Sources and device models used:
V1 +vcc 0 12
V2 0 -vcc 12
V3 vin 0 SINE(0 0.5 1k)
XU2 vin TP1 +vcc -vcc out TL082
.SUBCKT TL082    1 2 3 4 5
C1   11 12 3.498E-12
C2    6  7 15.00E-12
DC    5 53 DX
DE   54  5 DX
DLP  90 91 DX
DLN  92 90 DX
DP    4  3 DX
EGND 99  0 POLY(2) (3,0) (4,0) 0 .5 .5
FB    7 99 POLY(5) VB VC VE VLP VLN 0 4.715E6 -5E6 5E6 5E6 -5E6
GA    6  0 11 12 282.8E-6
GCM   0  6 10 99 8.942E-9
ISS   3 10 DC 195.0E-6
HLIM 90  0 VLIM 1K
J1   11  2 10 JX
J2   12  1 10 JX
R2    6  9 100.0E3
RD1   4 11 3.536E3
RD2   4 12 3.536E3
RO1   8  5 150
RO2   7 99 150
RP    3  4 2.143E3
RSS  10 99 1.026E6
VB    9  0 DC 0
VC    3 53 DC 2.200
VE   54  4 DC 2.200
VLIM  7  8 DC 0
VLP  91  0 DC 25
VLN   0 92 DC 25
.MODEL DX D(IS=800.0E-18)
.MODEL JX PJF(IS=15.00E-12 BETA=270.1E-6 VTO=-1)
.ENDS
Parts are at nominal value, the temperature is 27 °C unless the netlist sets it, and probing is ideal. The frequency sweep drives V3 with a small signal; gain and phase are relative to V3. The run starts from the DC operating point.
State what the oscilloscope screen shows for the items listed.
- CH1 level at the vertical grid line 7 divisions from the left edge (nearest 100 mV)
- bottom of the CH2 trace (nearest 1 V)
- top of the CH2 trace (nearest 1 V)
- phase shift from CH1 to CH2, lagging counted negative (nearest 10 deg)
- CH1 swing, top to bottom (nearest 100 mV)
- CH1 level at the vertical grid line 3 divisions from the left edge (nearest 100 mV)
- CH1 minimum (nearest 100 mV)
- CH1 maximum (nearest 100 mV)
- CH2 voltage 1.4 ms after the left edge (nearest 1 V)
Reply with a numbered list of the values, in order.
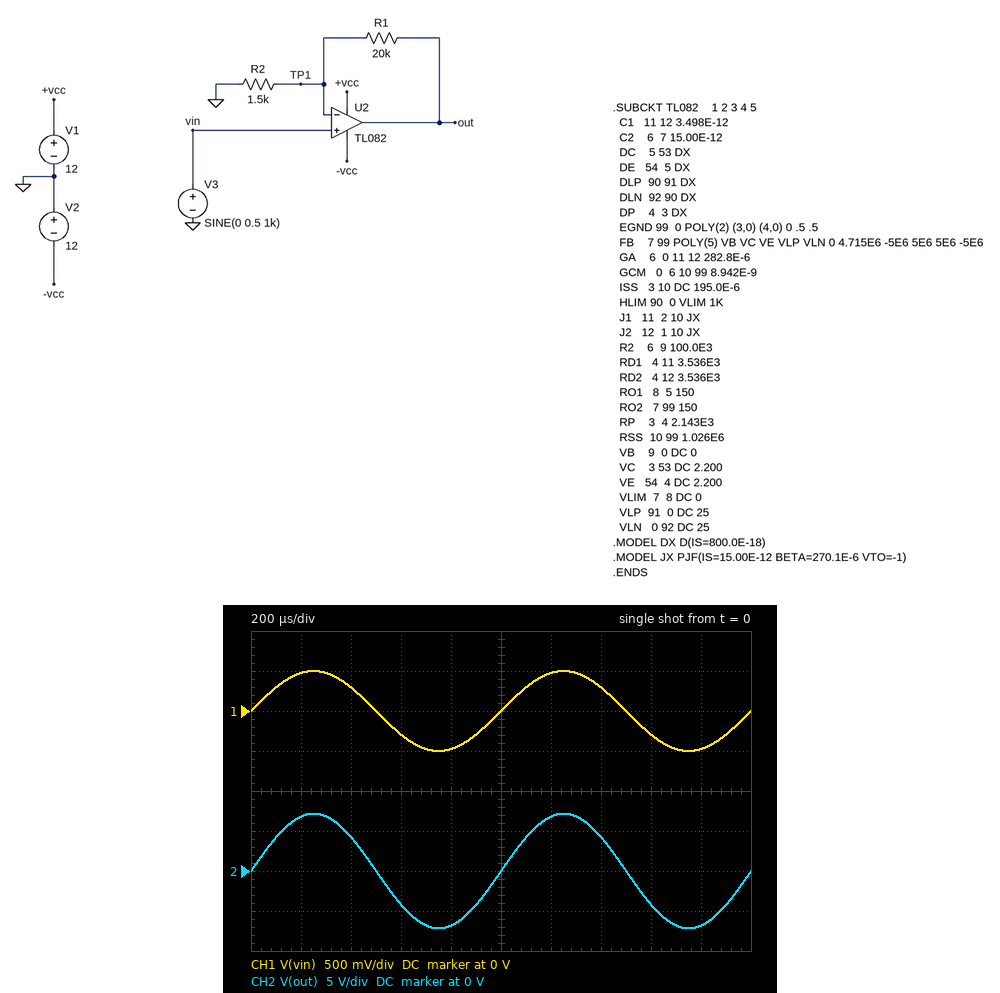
1. 300 mV
2. -7 V
3. 7 V
4. 0 deg
5. 1.0 V
6. -300 mV
7. -500 mV
8. 500 mV
9. 4 V
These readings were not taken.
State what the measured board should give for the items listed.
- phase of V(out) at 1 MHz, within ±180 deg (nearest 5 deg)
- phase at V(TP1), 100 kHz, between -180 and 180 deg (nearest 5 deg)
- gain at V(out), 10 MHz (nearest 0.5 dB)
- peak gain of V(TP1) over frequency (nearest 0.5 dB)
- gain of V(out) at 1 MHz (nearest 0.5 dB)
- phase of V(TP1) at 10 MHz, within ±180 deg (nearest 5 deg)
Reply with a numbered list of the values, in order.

1. -85 deg
2. -25 deg
3. -14.5 dB
4. 0 dB
5. 10.5 dB
6. -145 deg
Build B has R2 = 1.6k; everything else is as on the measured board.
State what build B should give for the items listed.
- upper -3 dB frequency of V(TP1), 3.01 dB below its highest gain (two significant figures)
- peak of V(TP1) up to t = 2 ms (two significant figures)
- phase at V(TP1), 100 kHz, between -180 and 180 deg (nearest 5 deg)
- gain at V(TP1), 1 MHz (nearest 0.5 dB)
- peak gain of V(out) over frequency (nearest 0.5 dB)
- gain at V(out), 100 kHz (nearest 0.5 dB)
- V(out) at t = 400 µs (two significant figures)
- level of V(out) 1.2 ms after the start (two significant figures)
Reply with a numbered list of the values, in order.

1. 260 kHz
2. 500 mV
3. -20 deg
4. -12.0 dB
5. 22.5 dB
6. 22.0 dB
7. 4.0 V
8. 6.4 V
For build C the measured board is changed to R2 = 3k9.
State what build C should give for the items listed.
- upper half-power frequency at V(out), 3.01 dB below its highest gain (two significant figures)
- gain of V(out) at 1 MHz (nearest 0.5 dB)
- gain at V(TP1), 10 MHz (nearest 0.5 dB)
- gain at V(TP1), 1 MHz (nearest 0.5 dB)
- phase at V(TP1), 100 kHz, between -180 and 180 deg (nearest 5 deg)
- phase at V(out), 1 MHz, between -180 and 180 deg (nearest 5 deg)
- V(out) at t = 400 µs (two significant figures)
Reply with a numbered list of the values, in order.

1. 610 kHz
2. 10.0 dB
3. -30.0 dB
4. -5.5 dB
5. -10 deg
6. -70 deg
7. 1.8 V
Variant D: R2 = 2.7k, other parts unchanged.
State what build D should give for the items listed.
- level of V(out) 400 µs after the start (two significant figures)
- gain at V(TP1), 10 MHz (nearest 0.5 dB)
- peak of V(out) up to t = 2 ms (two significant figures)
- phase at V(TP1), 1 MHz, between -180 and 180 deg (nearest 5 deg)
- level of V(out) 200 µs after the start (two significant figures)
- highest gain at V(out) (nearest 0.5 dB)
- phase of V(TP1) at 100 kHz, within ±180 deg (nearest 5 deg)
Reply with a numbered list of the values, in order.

1. 2.5 V
2. -33.0 dB
3. 4.2 V
4. -75 deg
5. 4.0 V
6. 18.5 dB
7. -15 deg
